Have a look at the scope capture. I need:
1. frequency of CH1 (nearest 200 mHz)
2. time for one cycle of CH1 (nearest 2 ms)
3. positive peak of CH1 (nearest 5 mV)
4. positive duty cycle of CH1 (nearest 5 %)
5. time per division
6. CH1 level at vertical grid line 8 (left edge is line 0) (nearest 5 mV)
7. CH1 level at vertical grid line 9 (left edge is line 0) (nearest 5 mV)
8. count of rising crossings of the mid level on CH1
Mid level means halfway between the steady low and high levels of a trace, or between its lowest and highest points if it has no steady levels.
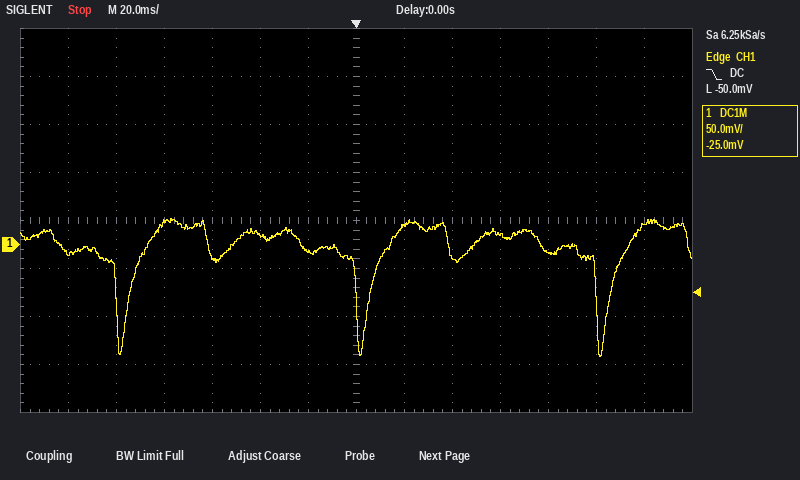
10.0 Hz
100 ms
25 mV
95 %
20 ms
20 mV
-15 mV
3
